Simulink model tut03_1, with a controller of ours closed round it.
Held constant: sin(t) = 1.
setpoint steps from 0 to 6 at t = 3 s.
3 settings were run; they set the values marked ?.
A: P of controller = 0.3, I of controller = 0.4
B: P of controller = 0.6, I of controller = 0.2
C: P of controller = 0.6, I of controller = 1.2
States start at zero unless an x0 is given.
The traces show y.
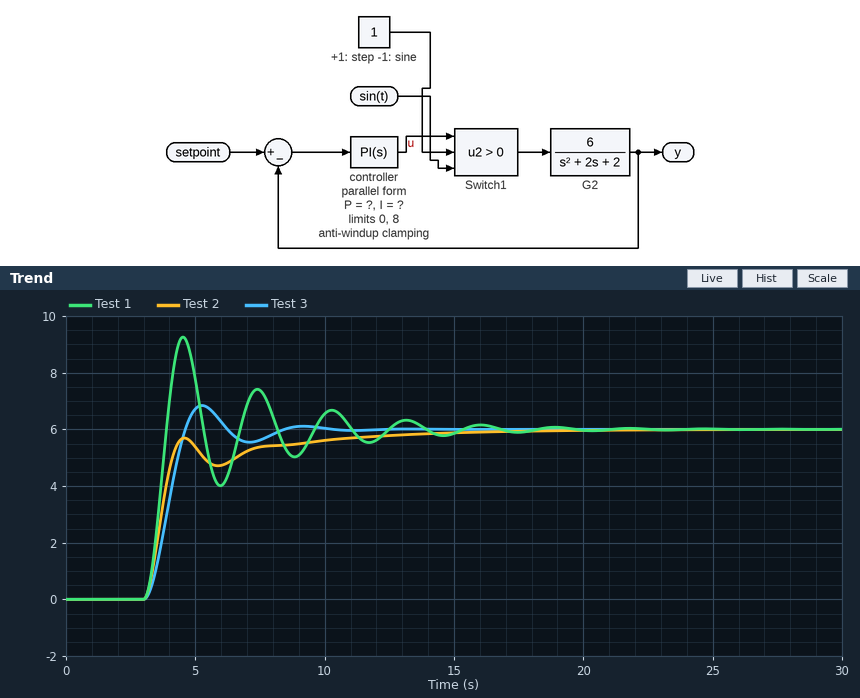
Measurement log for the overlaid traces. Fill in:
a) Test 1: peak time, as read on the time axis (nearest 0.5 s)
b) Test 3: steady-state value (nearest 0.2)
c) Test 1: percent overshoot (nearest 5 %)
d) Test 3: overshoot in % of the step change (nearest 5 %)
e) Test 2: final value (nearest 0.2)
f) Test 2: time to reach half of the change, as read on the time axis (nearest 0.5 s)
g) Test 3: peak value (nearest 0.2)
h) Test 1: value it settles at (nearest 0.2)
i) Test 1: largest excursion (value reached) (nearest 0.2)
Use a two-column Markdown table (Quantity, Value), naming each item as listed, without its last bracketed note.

| Quantity | Value |
|---|---|
| Test 1: peak time, as read on the time axis | 4.5 s |
| Test 3: steady-state value | 6.0 |
| Test 1: percent overshoot | 55 % |
| Test 3: overshoot in % of the step change | 15 % |
| Test 2: final value | 6.0 |
| Test 2: time to reach half of the change, as read on the time axis | 3.5 s |
| Test 3: peak value | 6.8 |
| Test 1: value it settles at | 6.0 |
| Test 1: largest excursion (value reached) | 9.2 |
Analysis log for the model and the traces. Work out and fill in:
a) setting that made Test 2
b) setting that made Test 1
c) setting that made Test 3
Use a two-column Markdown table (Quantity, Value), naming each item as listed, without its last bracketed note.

| Quantity | Value |
|---|---|
| setting that made Test 2 | B |
| setting that made Test 1 | C |
| setting that made Test 3 | A |
